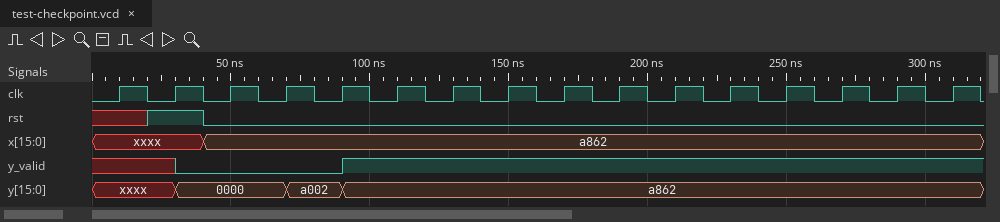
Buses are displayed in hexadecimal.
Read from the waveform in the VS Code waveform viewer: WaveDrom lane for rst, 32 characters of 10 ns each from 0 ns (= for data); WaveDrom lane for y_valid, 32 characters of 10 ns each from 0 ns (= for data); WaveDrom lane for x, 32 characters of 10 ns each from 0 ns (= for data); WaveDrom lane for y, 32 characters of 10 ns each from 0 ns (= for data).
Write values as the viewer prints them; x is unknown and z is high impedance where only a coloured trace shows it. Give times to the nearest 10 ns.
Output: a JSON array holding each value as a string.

["{name: 'rst', wave: 'x.1.0...........................'}", "{name: 'y_valid', wave: 'x..0.....1......................'}", "{name: 'x', wave: 'x...=...........................', data: 'a862'}", "{name: 'y', wave: 'x..=...=.=......................', data: '0000 a002 a862'}"]
